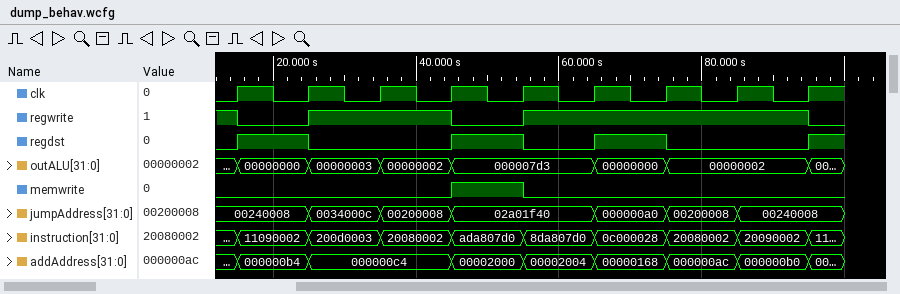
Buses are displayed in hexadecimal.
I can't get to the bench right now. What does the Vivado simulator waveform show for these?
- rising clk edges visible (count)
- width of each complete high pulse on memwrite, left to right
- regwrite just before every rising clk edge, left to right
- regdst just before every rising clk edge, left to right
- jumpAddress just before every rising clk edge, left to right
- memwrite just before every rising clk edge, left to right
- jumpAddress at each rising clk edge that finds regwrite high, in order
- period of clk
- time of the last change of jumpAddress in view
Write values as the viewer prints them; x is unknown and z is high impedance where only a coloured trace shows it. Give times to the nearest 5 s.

9
10 s
1 0 1 1 0 1 1 1 1
0 1 0 0 1 0 1 0 0
00240008, 00240008, 0034000c, 00200008, 02a01f40, 02a01f40, 000000a0, 00200008, 00240008
0 0 0 0 1 0 0 0 0
00240008, 0034000c, 00200008, 02a01f40, 000000a0, 00200008, 00240008
10 s
85 s
